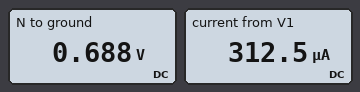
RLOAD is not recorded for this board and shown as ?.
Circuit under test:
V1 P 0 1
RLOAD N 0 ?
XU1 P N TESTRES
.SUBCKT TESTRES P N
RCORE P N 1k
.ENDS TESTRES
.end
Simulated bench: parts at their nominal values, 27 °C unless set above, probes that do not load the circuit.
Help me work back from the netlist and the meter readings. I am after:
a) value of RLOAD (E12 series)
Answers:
2.2 kΩ
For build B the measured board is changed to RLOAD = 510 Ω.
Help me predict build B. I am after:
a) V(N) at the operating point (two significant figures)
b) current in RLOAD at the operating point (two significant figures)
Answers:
340 mV
660 µA
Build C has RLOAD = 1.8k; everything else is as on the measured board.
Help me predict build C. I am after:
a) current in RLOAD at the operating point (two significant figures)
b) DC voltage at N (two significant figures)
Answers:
360 µA
640 mV
